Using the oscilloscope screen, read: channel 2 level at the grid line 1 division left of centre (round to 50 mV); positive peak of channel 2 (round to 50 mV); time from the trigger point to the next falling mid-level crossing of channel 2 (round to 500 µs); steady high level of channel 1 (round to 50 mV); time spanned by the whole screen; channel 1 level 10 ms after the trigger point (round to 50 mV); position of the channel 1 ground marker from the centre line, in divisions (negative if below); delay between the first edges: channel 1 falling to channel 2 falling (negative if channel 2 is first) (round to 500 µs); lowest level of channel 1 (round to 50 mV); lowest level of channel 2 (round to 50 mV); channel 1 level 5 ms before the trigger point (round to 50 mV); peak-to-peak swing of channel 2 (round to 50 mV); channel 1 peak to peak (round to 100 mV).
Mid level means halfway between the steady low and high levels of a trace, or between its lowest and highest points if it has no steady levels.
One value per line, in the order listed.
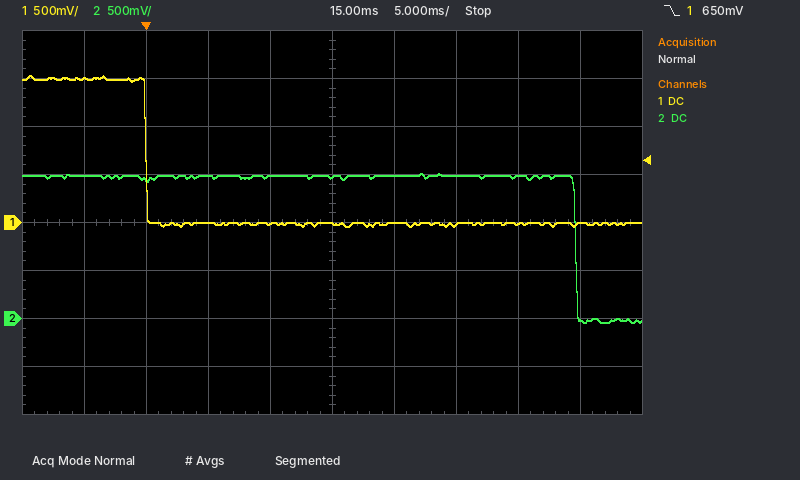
1.50 V
1.50 V
34.5 ms
1.50 V
50 ms
0 mV
0.0 div
+34.5 ms
-50 mV
-50 mV
1.50 V
1.55 V
1.60 V
